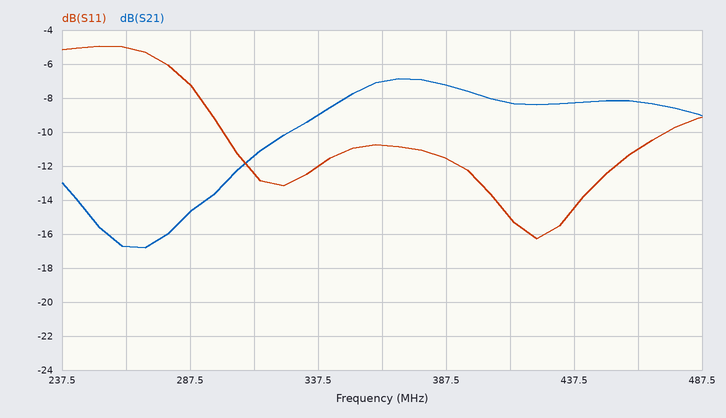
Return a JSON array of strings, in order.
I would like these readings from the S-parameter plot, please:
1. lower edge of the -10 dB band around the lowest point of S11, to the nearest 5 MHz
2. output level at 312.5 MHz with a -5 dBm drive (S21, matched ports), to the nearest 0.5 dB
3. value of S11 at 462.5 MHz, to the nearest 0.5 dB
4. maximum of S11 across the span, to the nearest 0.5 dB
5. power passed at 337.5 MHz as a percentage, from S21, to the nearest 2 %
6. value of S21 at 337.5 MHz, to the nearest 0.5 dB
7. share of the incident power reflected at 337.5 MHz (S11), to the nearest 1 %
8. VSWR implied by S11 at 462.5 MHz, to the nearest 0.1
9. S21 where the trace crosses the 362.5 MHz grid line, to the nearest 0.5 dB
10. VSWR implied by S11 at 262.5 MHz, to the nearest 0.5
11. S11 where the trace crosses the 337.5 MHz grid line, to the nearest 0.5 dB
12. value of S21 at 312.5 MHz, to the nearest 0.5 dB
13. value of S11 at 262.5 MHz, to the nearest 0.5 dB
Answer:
["300 MHz", "-16.5 dBm", "-11.0 dB", "-5.0 dB", "12 %", "-9.0 dB", "6 %", "1.8", "-7.0 dB", "3.5", "-12.0 dB", "-11.5 dB", "-5.0 dB"]
